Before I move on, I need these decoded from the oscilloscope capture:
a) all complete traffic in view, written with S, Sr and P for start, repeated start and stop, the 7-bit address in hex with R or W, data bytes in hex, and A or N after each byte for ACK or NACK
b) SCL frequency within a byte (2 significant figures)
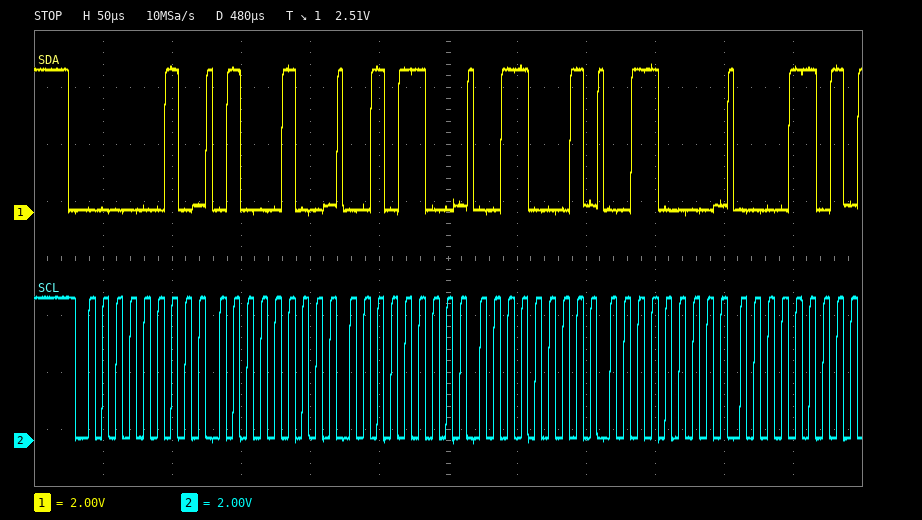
S 01W A 44 A 2C A 31 A 30 A 0D A
100 kHz
